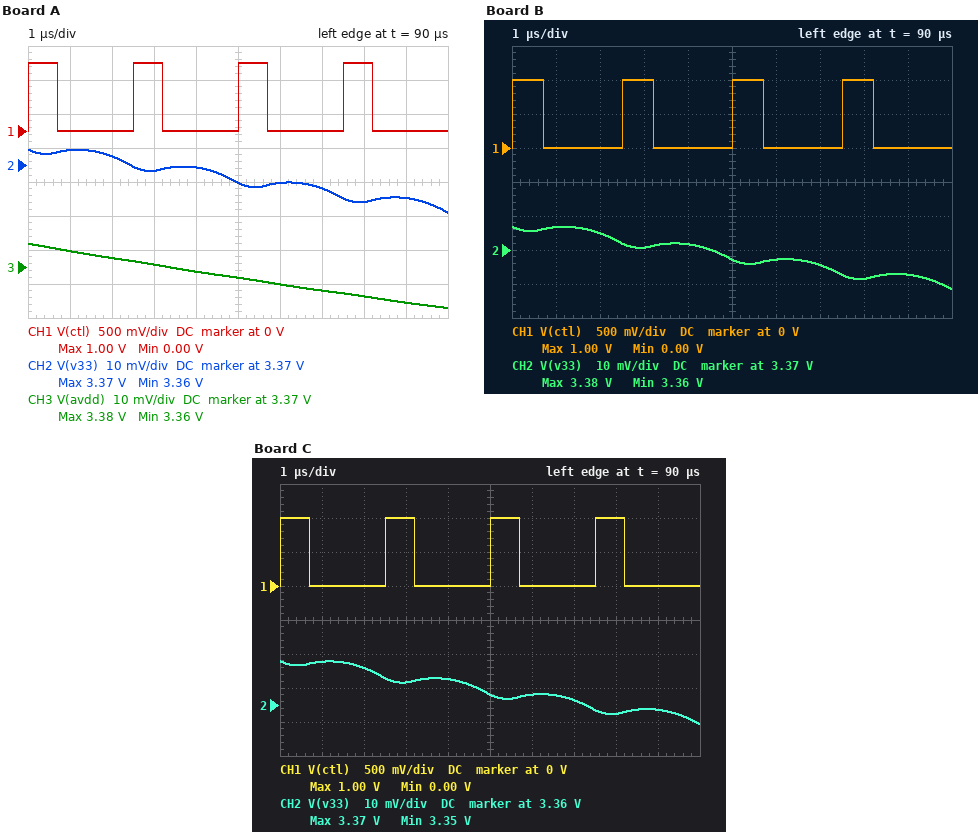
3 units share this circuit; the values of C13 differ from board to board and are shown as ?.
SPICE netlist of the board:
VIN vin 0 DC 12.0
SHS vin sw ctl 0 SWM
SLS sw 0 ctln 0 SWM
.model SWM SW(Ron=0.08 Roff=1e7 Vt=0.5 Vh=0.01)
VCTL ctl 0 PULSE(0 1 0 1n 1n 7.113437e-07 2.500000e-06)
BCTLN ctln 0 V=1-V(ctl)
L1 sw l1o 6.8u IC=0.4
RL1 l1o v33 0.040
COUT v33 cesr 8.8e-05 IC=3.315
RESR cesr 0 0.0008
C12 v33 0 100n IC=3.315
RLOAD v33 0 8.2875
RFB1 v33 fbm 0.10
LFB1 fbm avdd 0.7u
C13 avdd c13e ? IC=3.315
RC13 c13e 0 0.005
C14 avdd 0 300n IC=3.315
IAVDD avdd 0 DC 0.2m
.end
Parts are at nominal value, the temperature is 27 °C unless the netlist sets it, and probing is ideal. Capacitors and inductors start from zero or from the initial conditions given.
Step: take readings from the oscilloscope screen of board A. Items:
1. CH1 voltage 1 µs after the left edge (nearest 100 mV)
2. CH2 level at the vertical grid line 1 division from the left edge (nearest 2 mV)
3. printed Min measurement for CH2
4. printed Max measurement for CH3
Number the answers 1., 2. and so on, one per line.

1. 0 V
2. 3.374 V
3. 3.36 V
4. 3.38 V
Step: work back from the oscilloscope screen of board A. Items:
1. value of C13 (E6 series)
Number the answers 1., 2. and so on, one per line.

1. 4.7 µF
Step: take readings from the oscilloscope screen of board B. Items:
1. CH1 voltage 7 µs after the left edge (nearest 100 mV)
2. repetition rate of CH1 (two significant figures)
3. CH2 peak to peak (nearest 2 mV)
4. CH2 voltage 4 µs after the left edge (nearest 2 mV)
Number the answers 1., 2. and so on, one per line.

1. 0 V
2. 400 kHz
3. 18 mV
4. 3.372 V
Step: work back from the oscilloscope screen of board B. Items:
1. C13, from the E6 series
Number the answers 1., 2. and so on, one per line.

1. 6.8 µF
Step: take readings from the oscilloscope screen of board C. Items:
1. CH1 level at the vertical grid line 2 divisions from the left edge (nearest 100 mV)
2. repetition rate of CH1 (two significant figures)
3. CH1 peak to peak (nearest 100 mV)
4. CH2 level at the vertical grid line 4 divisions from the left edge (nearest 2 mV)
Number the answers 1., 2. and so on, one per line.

1. 0 V
2. 400 kHz
3. 1.0 V
4. 3.368 V
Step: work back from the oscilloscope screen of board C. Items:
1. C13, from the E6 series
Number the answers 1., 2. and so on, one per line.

1. 3.3 µF
